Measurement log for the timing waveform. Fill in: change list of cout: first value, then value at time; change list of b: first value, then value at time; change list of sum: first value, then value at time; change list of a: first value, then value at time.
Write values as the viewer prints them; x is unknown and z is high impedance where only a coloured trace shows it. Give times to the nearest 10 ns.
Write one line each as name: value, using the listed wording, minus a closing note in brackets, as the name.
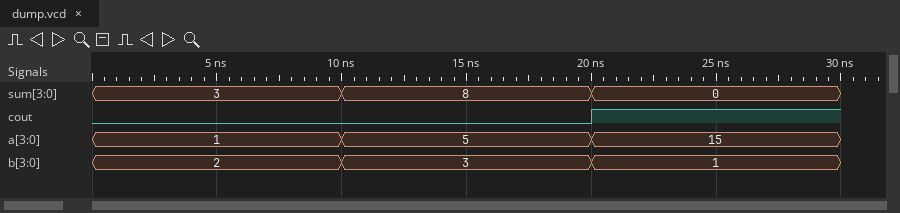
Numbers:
change list of cout: first value, then value at time: 0, 1 at 20 ns
change list of b: first value, then value at time: 2, 3 at 10 ns, 1 at 20 ns
change list of sum: first value, then value at time: 3, 8 at 10 ns, 0 at 20 ns
change list of a: first value, then value at time: 1, 5 at 10 ns, 15 at 20 ns
